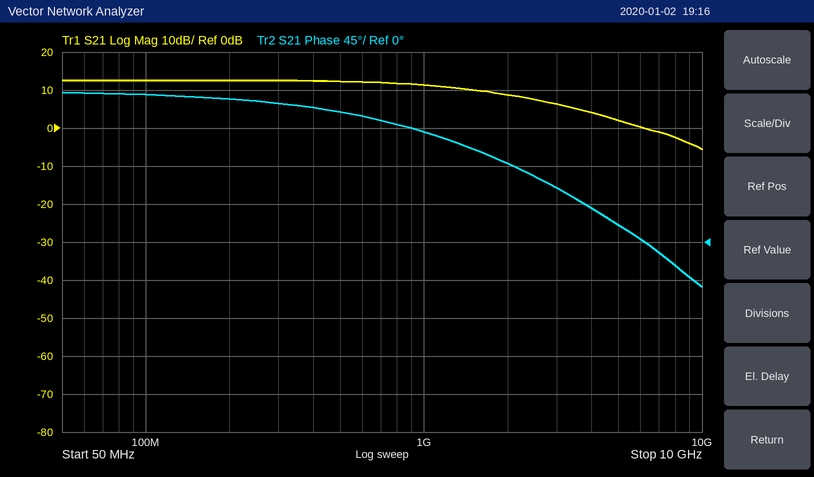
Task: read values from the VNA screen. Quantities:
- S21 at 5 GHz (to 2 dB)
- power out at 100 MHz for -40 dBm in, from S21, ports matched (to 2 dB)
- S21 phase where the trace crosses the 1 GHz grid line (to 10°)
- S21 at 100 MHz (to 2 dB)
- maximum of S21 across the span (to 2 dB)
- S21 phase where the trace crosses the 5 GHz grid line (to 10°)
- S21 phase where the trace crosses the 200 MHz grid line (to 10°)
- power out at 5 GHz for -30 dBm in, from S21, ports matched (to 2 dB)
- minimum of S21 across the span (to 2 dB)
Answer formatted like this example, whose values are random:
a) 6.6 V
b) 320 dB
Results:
a) 2 dB
b) -28 dBm
c) 130°
d) 12 dB
e) 12 dB
f) 20°
g) 170°
h) -28 dBm
i) -6 dB
